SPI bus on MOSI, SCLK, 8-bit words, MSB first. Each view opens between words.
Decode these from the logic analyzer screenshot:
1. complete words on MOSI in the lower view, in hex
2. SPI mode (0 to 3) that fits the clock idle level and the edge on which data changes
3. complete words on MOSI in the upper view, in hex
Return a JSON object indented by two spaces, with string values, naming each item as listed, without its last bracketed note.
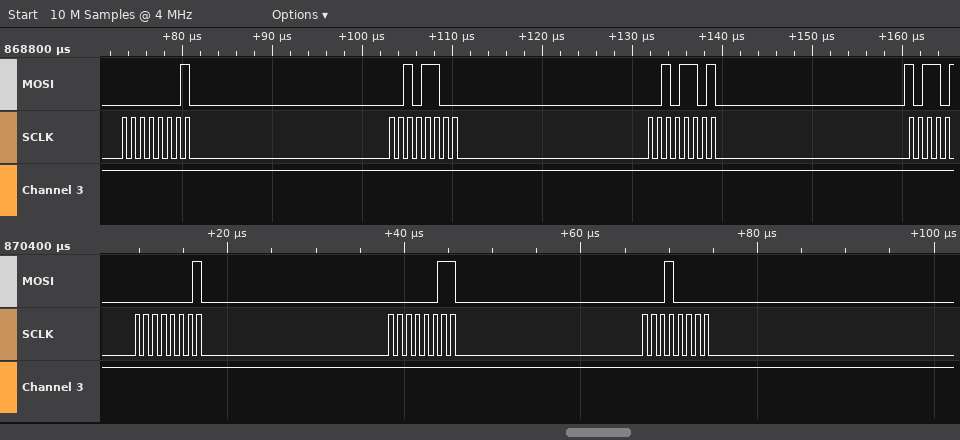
{
  "complete words on MOSI in the lower view, in hex": "01, 03, 10",
  "SPI mode (0 to 3) that fits the clock idle level and the edge on which data changes": "0",
  "complete words on MOSI in the upper view, in hex": "01, 2C, 2D"
}
